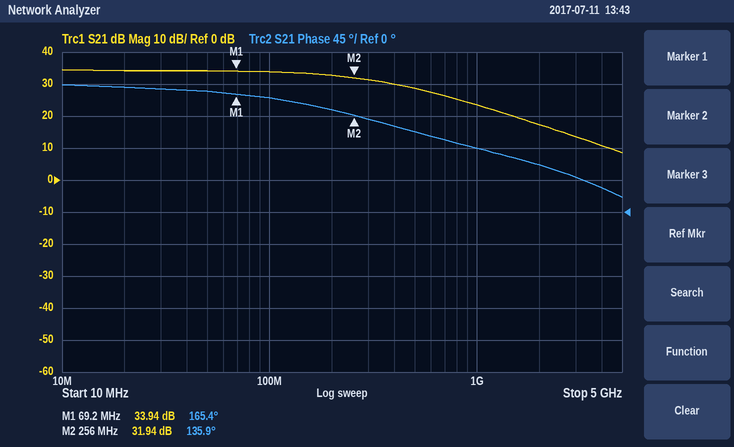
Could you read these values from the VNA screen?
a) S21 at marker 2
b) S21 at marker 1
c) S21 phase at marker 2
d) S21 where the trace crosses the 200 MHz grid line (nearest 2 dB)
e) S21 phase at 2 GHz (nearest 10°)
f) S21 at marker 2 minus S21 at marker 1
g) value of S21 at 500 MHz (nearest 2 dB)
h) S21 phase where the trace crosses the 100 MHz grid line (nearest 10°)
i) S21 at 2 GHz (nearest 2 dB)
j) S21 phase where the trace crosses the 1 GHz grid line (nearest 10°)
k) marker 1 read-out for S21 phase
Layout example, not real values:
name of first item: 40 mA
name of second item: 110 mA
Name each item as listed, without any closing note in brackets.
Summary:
S21 at marker 2: 31.94 dB
S21 at marker 1: 33.94 dB
S21 phase at marker 2: 135.9°
S21 where the trace crosses the 200 MHz grid line: 32 dB
S21 phase at 2 GHz: 70°
S21 at marker 2 minus S21 at marker 1: -2.00 dB
value of S21 at 500 MHz: 28 dB
S21 phase where the trace crosses the 100 MHz grid line: 160°
S21 at 2 GHz: 18 dB
S21 phase where the trace crosses the 1 GHz grid line: 90°
marker 1 read-out for S21 phase: 165.4°
